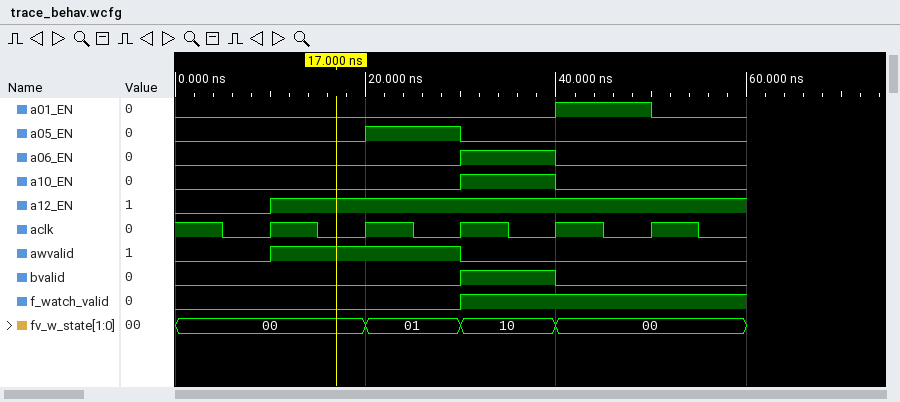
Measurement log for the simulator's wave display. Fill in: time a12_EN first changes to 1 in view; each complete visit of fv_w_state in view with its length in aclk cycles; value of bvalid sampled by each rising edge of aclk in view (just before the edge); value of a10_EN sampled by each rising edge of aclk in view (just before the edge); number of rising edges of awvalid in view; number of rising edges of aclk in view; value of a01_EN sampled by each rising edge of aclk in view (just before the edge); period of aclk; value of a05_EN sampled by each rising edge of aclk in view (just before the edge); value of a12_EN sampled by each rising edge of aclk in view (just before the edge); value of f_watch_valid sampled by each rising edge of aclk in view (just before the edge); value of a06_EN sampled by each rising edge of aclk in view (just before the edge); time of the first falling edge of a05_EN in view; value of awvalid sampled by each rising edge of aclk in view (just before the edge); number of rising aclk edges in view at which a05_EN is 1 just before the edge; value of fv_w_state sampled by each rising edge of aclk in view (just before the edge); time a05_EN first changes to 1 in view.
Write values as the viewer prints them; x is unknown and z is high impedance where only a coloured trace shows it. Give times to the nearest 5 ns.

10 ns
01: 1, 10: 1
0 0 0 1 0
0 0 0 1 0
1
5
0 0 0 0 1
10 ns
0 0 1 0 0
0 1 1 1 1
0 0 0 1 1
0 0 0 1 0
30 ns
0 1 1 0 0
1
00, 00, 01, 10, 00
20 ns
